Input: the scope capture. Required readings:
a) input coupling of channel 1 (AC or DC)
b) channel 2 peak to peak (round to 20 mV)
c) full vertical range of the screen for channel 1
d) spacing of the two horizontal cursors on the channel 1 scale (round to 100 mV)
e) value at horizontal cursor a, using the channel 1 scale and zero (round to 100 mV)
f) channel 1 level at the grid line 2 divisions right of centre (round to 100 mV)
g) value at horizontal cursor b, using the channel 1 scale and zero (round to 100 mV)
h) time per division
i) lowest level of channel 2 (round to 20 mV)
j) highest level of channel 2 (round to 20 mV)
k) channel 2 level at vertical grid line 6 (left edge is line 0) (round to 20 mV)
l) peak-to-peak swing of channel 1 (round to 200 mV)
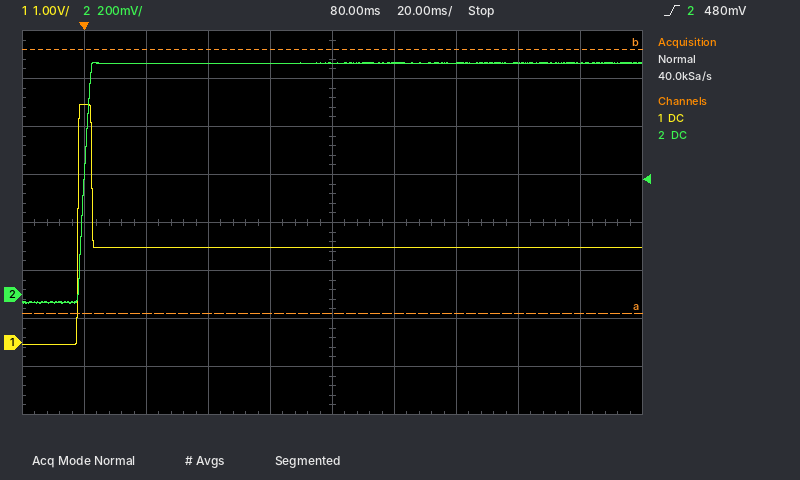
DC
1.00 V
8 V
5.5 V
600 mV
2.0 V
6.1 V
20 ms
-40 mV
960 mV
960 mV
5.0 V
